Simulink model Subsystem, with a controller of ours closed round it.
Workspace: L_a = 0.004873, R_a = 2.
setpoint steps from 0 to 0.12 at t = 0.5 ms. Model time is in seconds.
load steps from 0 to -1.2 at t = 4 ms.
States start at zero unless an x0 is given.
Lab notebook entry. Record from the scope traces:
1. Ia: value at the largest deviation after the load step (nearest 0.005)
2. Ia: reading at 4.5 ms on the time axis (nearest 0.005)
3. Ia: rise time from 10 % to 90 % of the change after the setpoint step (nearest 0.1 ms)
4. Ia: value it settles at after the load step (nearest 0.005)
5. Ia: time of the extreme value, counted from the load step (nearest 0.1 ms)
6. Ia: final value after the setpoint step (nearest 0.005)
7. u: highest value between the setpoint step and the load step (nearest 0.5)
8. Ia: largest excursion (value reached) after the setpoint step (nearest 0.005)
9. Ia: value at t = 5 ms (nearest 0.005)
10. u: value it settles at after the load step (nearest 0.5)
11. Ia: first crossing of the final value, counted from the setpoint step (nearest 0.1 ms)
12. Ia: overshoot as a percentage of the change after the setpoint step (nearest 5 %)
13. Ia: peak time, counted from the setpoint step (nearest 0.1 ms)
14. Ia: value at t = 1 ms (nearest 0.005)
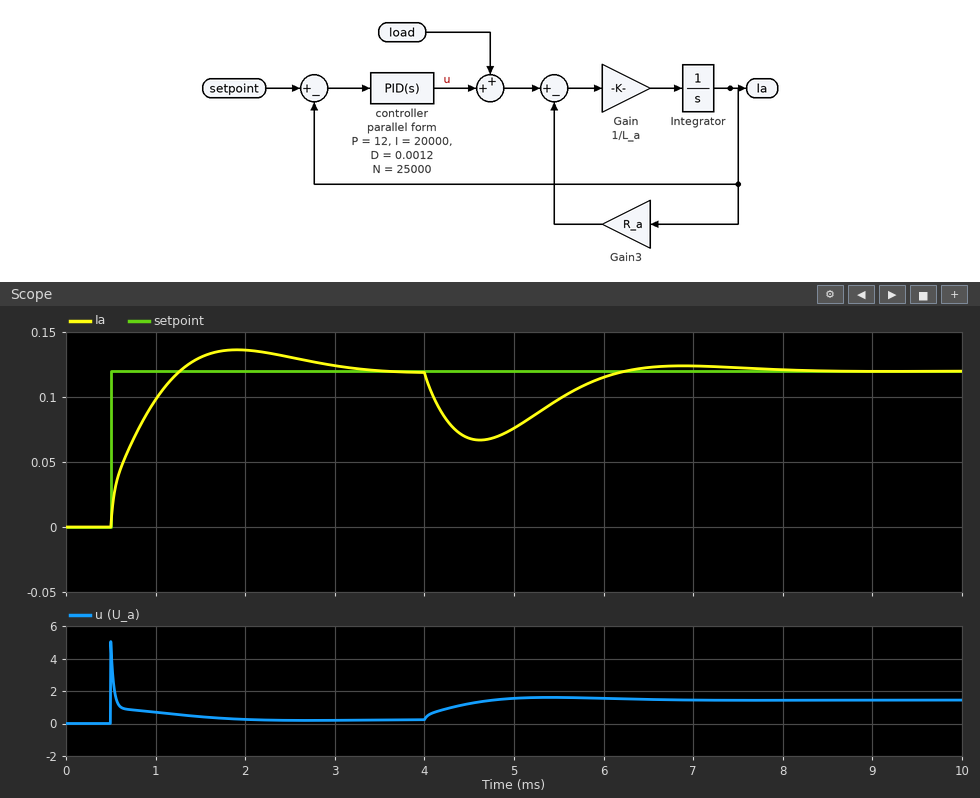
0.065
0.070
0.6 ms
0.120
0.6 ms
0.120
5.0
0.135
0.075
1.5
0.8 ms
15 %
1.4 ms
0.100
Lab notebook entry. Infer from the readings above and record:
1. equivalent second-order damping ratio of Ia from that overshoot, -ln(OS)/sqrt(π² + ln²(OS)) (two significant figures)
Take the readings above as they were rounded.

0.52
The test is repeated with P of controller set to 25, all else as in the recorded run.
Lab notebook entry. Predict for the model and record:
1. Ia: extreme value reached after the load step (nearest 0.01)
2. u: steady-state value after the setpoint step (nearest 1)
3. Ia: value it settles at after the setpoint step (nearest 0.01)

0.09
0
0.12
